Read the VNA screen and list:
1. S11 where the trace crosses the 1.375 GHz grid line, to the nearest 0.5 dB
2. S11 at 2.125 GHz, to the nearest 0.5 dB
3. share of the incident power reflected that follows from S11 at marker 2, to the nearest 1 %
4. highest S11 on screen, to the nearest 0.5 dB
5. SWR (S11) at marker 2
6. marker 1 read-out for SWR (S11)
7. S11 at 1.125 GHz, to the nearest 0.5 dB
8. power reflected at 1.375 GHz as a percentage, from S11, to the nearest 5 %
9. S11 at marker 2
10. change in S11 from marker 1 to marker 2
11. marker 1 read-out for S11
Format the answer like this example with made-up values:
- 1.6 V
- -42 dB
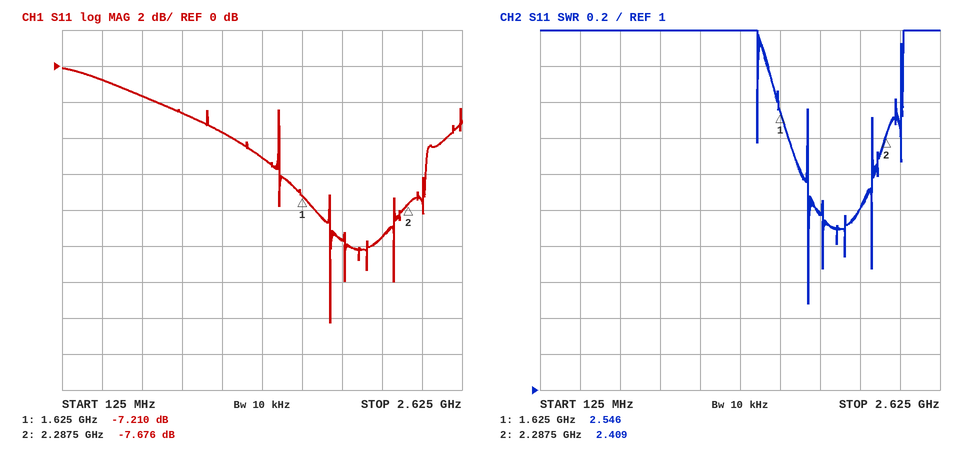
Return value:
- -5.0 dB
- -9.5 dB
- 17 %
- 0.0 dB
- 2.409
- 2.546
- -3.5 dB
- 30 %
- -7.676 dB
- -0.466 dB
- -7.210 dB
